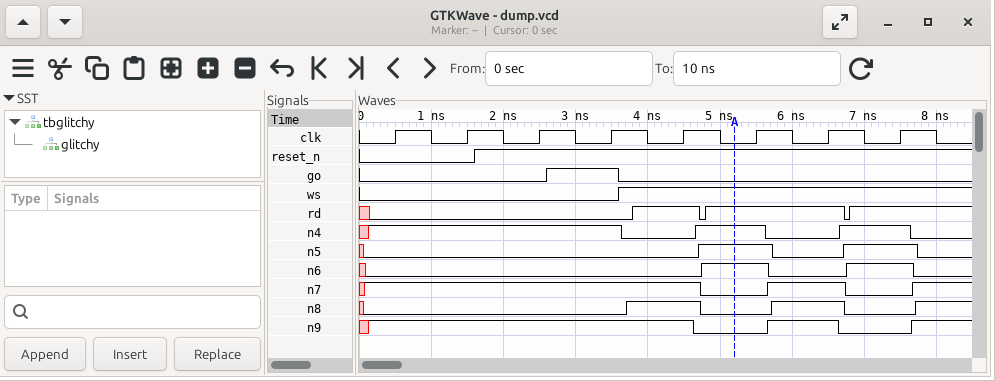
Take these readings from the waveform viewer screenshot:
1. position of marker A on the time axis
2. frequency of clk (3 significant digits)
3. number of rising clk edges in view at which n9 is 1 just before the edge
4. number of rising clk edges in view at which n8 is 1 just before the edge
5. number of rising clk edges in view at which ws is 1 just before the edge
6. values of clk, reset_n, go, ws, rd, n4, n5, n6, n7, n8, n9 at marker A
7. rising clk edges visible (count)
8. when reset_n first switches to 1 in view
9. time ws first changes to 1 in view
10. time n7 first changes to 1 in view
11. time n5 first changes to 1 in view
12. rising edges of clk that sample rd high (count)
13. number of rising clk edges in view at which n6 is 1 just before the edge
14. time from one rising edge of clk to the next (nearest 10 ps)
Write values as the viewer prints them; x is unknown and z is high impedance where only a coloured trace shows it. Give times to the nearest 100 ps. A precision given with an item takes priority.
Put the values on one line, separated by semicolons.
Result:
5200 ps; 1.00 GHz; 6; 2; 4; clk=0, reset_n=1, go=0, ws=1, rd=1, n4=1, n5=1, n6=1, n7=0, n8=0, n9=0; 8; 1600 ps; 3600 ps; 100 ps; 4700 ps; 4; 2; 1000 ps
